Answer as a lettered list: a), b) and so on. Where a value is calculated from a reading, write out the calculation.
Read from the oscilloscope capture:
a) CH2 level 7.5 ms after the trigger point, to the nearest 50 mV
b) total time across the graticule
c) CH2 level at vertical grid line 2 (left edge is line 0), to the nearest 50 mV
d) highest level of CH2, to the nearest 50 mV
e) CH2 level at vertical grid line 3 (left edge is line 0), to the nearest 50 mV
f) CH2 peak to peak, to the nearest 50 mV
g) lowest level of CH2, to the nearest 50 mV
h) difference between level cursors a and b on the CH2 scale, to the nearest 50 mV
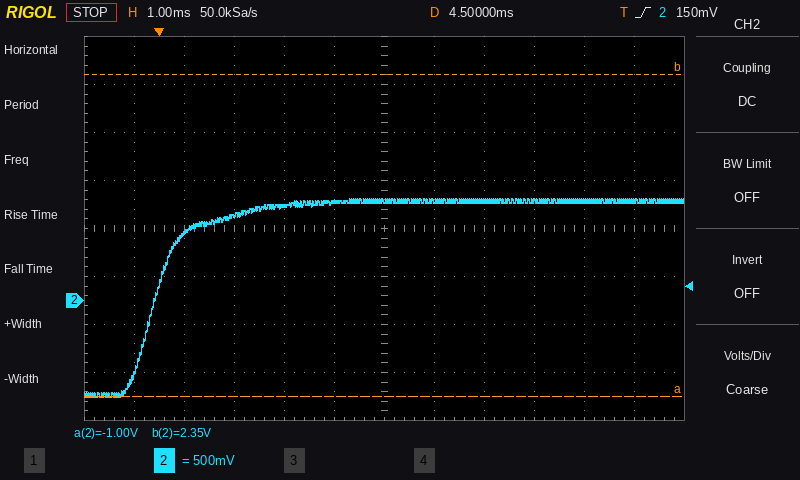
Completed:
a) 1.05 V
b) 12 ms
c) 700 mV
d) 1.05 V
e) 900 mV
f) 1.05 V − (-1.00 V) = 2.05 V
g) -1.00 V
h) 3.35 V
